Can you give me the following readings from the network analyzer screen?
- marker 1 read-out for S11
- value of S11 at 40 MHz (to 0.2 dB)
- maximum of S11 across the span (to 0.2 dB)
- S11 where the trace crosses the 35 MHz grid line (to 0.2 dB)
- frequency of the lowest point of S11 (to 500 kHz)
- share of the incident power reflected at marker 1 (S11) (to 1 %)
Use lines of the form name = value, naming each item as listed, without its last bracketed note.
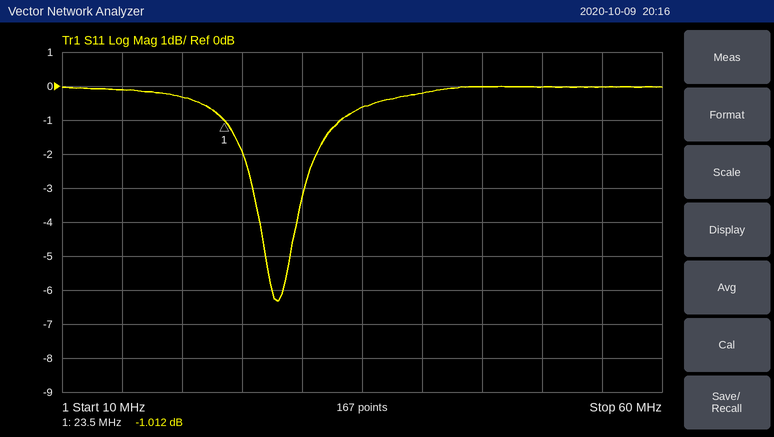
marker 1 read-out for S11 = -1.012 dB
value of S11 at 40 MHz = -0.2 dB
maximum of S11 across the span = 0.0 dB
S11 where the trace crosses the 35 MHz grid line = -0.6 dB
frequency of the lowest point of S11 = 28.0 MHz
share of the incident power reflected at marker 1 (S11) = 79 %
